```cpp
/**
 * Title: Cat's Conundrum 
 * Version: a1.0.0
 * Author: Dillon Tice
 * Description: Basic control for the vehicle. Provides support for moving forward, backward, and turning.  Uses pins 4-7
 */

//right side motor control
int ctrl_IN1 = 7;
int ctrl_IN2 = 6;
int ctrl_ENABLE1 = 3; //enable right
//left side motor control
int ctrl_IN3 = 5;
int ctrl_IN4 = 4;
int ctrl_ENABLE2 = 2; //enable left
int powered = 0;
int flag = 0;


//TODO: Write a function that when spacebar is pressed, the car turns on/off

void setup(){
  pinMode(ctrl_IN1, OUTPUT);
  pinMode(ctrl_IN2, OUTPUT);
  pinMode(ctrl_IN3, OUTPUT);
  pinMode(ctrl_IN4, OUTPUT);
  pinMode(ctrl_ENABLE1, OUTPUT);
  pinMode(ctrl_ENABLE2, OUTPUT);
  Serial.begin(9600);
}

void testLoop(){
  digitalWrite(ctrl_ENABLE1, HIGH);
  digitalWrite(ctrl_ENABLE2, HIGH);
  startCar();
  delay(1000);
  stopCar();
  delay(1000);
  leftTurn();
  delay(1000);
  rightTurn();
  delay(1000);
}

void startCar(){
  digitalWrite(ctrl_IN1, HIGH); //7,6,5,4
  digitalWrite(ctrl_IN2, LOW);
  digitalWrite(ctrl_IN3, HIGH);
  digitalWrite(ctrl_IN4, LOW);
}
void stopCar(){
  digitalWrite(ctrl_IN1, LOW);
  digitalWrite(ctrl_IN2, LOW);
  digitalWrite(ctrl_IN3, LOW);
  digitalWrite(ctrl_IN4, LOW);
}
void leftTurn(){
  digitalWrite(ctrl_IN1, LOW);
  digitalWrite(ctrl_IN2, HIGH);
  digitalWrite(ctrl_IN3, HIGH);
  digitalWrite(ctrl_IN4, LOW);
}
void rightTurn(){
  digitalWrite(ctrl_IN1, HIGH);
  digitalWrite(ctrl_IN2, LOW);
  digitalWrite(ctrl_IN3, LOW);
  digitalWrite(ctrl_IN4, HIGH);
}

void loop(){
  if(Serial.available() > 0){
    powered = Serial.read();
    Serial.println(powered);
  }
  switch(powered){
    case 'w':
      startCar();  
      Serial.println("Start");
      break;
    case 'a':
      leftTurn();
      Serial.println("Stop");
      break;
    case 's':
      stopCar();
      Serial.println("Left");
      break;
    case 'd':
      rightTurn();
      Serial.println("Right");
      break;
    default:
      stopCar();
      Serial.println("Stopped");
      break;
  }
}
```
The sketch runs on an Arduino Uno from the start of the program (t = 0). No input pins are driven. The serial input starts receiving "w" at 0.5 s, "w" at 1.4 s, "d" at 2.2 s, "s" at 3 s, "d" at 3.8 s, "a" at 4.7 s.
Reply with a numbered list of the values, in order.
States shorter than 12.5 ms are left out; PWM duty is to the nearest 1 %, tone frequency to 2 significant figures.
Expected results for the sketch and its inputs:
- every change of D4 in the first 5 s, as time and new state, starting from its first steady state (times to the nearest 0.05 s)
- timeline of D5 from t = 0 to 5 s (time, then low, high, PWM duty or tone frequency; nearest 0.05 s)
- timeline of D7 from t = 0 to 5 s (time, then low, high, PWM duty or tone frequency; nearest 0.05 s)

1. 0 s low; 2.2 s high; 3 s low; 3.8 s high; 4.7 s low
2. 0 s low; 0.5 s high; 2.2 s low; 4.7 s high
3. 0 s low; 0.5 s high; 3 s low; 3.8 s high; 4.7 s low
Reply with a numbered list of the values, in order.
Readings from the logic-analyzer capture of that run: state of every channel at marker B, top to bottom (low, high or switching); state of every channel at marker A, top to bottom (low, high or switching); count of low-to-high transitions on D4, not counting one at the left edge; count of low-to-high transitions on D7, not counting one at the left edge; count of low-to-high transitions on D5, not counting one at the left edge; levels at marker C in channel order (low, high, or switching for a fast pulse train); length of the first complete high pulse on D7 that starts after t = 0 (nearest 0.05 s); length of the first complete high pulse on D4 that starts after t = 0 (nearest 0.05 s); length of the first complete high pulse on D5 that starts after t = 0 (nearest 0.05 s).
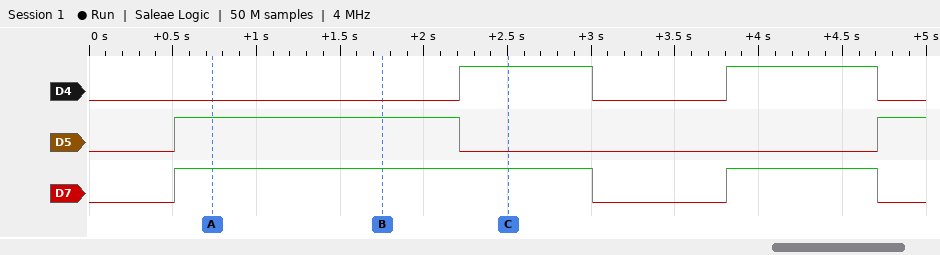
1. D4 low, D5 high, D7 high
2. D4 low, D5 high, D7 high
3. 2
4. 2
5. 2
6. D4 high, D5 low, D7 high
7. 2.50 s
8. 0.80 s
9. 1.70 s
